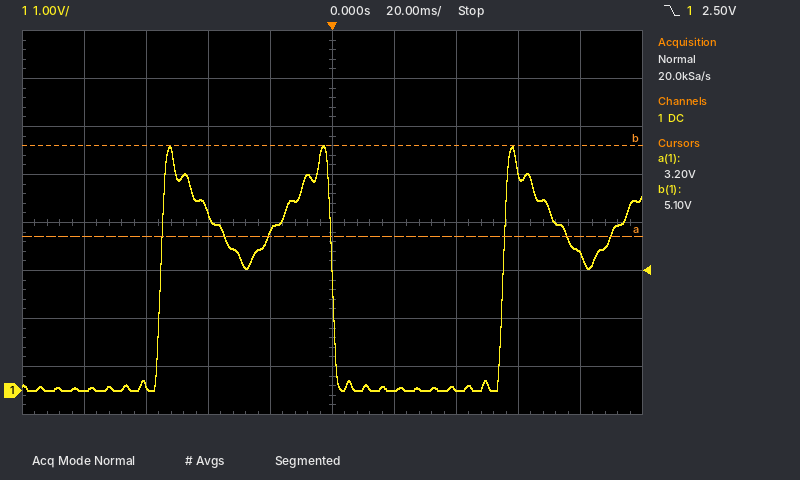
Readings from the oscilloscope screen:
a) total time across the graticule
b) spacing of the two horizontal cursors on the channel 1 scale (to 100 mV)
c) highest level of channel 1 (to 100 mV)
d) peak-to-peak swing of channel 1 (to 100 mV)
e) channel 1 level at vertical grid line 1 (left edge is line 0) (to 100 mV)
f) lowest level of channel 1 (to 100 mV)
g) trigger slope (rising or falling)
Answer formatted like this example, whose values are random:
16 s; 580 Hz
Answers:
200 ms; 1.9 V; 5.1 V; 5.1 V; 0.0 V; 0.0 V; falling
